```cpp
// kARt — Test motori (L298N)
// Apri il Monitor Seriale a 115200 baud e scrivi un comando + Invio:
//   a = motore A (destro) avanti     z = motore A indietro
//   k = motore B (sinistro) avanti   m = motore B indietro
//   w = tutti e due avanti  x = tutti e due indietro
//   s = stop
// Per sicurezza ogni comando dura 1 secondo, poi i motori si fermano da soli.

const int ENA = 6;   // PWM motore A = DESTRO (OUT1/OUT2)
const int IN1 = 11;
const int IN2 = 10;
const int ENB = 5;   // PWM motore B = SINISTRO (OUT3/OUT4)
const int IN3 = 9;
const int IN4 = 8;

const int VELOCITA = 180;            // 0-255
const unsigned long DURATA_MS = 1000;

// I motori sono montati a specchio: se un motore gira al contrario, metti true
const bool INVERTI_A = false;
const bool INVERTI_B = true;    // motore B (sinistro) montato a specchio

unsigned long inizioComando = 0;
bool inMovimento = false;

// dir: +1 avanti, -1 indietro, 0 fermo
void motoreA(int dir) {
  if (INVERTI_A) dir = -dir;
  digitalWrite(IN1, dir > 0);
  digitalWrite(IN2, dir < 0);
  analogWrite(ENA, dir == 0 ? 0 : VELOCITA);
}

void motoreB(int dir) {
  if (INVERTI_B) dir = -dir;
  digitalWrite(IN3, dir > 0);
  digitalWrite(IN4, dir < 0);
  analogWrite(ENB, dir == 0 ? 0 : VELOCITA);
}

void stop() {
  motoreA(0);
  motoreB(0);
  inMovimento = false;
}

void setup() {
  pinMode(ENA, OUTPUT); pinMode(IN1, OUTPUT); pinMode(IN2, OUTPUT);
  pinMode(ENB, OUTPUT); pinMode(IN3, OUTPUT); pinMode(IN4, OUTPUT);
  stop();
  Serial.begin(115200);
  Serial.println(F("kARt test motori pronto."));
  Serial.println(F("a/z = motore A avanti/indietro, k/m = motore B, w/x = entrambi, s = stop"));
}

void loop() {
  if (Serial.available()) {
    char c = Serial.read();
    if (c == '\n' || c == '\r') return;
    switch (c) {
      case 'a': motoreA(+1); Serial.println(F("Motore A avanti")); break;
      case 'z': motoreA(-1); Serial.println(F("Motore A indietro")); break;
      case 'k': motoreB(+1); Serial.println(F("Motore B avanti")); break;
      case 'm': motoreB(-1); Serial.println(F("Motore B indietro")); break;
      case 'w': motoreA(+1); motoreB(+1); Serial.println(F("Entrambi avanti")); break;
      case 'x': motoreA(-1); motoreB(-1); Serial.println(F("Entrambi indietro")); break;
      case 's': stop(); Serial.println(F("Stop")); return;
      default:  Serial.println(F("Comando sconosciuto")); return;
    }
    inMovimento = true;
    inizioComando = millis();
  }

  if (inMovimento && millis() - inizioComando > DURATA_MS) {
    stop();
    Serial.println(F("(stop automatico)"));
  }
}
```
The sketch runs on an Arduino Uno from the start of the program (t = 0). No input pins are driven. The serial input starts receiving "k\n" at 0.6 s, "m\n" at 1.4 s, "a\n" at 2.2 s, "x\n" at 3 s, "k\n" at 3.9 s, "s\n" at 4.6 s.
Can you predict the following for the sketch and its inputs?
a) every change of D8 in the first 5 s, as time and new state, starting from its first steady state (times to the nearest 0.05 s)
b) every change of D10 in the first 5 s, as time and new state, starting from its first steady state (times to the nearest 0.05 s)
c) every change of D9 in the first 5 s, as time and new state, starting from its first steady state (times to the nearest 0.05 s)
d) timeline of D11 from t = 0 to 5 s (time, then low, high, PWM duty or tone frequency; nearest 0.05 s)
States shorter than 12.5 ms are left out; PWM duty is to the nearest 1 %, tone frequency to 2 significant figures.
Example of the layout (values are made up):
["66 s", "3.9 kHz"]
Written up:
["0 s low; 0.6 s high; 1.4 s low; 3.9 s high; 4.6 s low", "0 s low; 3 s high; 4.6 s low", "0 s low; 1.4 s high; 3.9 s low", "0 s low; 2.2 s high; 3 s low"]
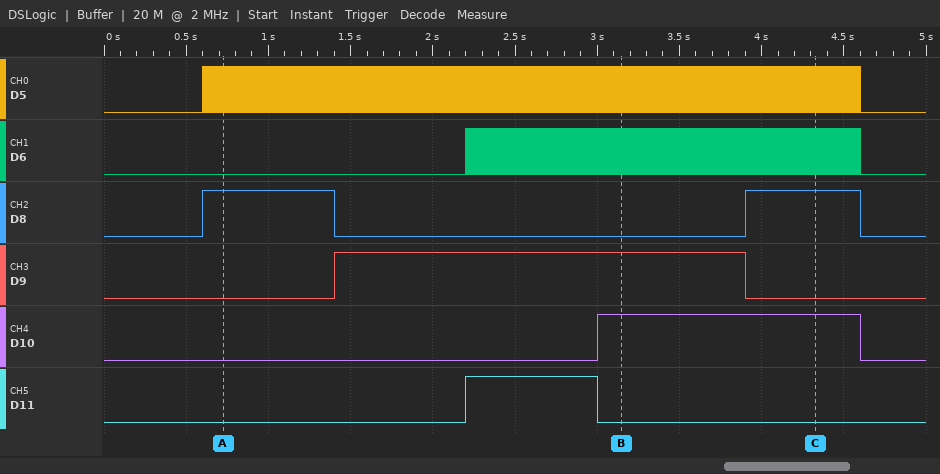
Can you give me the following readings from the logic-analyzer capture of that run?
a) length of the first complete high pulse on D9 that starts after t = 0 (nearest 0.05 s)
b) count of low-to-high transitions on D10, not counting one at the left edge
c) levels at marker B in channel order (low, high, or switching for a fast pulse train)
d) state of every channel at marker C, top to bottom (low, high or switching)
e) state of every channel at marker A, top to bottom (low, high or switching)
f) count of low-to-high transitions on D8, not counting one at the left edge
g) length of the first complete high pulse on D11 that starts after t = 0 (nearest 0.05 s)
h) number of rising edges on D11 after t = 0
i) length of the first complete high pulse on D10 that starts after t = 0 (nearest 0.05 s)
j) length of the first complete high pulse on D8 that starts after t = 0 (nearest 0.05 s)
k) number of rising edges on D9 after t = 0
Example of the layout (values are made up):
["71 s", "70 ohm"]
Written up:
["2.50 s", "1", "D5 switching, D6 switching, D8 low, D9 high, D10 high, D11 low", "D5 switching, D6 switching, D8 high, D9 low, D10 high, D11 low", "D5 switching, D6 low, D8 high, D9 low, D10 low, D11 low", "2", "0.80 s", "1", "1.60 s", "0.80 s", "1"]
